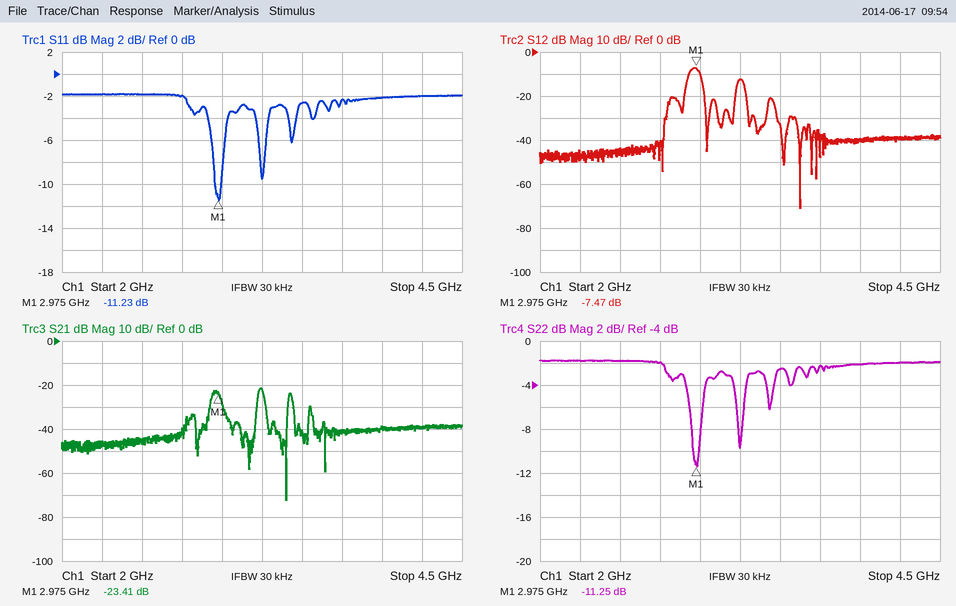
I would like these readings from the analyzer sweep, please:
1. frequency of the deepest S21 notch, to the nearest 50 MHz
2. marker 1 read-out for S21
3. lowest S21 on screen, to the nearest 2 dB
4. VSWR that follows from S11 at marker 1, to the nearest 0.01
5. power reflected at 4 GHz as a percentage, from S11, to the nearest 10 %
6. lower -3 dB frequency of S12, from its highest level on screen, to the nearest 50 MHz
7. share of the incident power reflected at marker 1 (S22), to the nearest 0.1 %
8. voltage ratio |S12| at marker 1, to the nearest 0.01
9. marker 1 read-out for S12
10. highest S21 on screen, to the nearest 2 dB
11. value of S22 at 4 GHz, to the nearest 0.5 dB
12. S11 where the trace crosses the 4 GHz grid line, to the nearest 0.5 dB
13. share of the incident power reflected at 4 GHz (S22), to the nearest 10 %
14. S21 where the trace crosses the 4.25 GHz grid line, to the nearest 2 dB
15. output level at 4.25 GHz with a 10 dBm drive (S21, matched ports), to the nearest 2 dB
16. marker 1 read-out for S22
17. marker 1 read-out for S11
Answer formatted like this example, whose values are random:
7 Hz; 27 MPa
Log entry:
3.40 GHz; -23.41 dB; -72 dB; 1.76; 60 %; 2.95 GHz; 7.5 %; 0.42; -7.47 dB; -22 dB; -2.0 dB; -2.0 dB; 60 %; -40 dB; -30 dBm; -11.25 dB; -11.23 dB
